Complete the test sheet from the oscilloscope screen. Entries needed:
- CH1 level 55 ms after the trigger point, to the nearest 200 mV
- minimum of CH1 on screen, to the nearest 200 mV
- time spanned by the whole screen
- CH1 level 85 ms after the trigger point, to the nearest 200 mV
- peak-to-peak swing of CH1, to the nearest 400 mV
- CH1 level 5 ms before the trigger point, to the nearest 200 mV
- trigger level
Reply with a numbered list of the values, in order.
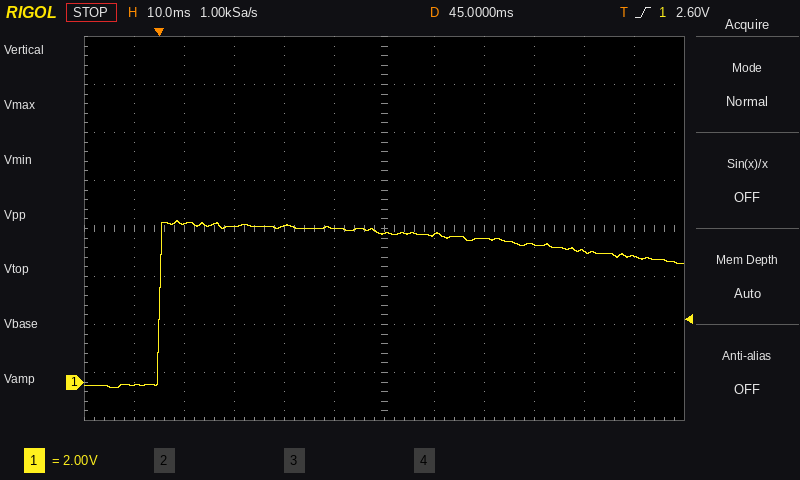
1. 6.2 V
2. -200 mV
3. 120 ms
4. 5.4 V
5. 6.8 V
6. -200 mV
7. 2.60 V
